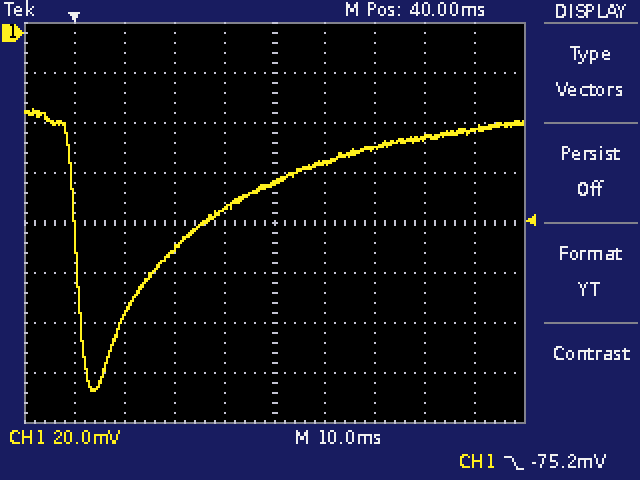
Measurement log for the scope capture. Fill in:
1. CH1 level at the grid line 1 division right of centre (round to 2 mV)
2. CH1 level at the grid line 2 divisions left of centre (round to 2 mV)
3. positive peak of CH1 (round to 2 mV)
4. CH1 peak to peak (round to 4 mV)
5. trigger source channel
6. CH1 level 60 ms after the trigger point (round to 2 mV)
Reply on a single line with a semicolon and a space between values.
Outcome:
-52 mV; -86 mV; -30 mV; 112 mV; CH1; -46 mV
